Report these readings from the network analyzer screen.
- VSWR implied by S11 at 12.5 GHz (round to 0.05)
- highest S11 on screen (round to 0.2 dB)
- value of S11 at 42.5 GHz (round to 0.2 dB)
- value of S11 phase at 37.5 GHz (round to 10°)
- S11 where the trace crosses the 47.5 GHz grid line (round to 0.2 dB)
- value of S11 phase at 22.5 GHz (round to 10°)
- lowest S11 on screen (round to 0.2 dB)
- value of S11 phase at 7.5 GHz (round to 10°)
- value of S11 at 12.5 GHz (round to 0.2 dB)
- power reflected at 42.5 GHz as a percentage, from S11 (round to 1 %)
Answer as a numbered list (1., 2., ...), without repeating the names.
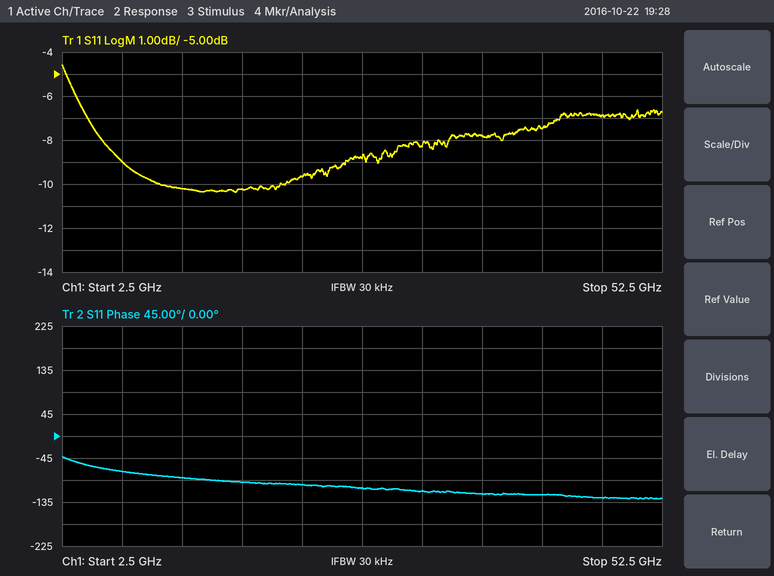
1. 1.90
2. -4.6 dB
3. -7.4 dB
4. -120°
5. -6.8 dB
6. -100°
7. -10.4 dB
8. -70°
9. -10.2 dB
10. 18 %
